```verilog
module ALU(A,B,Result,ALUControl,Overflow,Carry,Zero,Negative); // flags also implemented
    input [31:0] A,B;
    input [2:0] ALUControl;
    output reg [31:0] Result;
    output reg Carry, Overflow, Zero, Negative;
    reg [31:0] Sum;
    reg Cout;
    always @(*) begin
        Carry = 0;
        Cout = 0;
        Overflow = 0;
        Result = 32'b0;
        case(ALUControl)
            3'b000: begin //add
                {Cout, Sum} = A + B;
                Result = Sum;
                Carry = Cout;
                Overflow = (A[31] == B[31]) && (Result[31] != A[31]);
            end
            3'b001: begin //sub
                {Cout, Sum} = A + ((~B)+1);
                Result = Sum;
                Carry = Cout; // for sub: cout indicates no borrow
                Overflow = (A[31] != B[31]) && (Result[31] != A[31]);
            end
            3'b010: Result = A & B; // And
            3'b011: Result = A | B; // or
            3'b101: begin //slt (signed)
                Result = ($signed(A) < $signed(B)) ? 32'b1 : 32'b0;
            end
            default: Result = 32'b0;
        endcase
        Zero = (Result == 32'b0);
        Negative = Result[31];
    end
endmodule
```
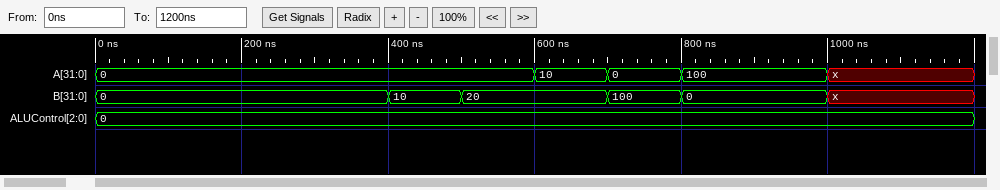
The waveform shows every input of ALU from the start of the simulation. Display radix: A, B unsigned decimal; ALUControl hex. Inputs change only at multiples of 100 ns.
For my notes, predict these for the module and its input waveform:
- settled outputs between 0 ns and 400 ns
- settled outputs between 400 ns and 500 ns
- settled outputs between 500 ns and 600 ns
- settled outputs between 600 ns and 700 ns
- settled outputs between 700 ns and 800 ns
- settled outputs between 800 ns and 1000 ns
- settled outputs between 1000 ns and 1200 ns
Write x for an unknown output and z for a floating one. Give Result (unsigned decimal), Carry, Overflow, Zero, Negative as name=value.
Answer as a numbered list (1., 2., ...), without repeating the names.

1. Result=0, Carry=0, Overflow=0, Zero=1, Negative=0
2. Result=10, Carry=0, Overflow=0, Zero=0, Negative=0
3. Result=20, Carry=0, Overflow=0, Zero=0, Negative=0
4. Result=30, Carry=0, Overflow=0, Zero=0, Negative=0
5. Result=100, Carry=0, Overflow=0, Zero=0, Negative=0
6. Result=100, Carry=0, Overflow=0, Zero=0, Negative=0
7. Result=x, Carry=x, Overflow=x, Zero=x, Negative=x
